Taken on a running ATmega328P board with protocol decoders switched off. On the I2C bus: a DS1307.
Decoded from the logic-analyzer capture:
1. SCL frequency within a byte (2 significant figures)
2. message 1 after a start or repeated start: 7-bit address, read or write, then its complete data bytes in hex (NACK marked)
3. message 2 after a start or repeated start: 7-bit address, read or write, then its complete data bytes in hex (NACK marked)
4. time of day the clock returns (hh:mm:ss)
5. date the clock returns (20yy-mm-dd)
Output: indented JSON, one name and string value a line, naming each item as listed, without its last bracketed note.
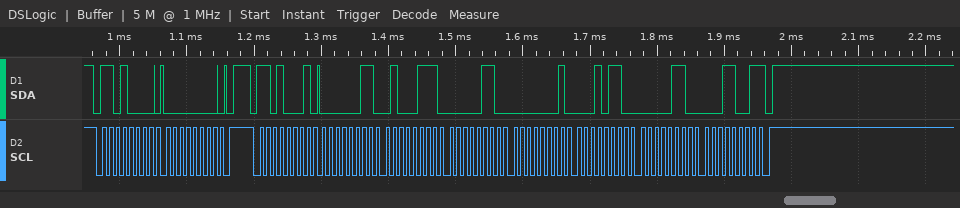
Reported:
{
  "SCL frequency within a byte": "100 kHz",
  "message 1 after a start or repeated start: 7-bit address, read or write, then its complete data bytes in hex": "0x68 write: 00",
  "message 2 after a start or repeated start: 7-bit address, read or write, then its complete data bytes in hex": "0x68 read: 03 47 06 01 16 06 19 NACK",
  "time of day the clock returns": "06:47:03",
  "date the clock returns": "2019-06-16"
}
